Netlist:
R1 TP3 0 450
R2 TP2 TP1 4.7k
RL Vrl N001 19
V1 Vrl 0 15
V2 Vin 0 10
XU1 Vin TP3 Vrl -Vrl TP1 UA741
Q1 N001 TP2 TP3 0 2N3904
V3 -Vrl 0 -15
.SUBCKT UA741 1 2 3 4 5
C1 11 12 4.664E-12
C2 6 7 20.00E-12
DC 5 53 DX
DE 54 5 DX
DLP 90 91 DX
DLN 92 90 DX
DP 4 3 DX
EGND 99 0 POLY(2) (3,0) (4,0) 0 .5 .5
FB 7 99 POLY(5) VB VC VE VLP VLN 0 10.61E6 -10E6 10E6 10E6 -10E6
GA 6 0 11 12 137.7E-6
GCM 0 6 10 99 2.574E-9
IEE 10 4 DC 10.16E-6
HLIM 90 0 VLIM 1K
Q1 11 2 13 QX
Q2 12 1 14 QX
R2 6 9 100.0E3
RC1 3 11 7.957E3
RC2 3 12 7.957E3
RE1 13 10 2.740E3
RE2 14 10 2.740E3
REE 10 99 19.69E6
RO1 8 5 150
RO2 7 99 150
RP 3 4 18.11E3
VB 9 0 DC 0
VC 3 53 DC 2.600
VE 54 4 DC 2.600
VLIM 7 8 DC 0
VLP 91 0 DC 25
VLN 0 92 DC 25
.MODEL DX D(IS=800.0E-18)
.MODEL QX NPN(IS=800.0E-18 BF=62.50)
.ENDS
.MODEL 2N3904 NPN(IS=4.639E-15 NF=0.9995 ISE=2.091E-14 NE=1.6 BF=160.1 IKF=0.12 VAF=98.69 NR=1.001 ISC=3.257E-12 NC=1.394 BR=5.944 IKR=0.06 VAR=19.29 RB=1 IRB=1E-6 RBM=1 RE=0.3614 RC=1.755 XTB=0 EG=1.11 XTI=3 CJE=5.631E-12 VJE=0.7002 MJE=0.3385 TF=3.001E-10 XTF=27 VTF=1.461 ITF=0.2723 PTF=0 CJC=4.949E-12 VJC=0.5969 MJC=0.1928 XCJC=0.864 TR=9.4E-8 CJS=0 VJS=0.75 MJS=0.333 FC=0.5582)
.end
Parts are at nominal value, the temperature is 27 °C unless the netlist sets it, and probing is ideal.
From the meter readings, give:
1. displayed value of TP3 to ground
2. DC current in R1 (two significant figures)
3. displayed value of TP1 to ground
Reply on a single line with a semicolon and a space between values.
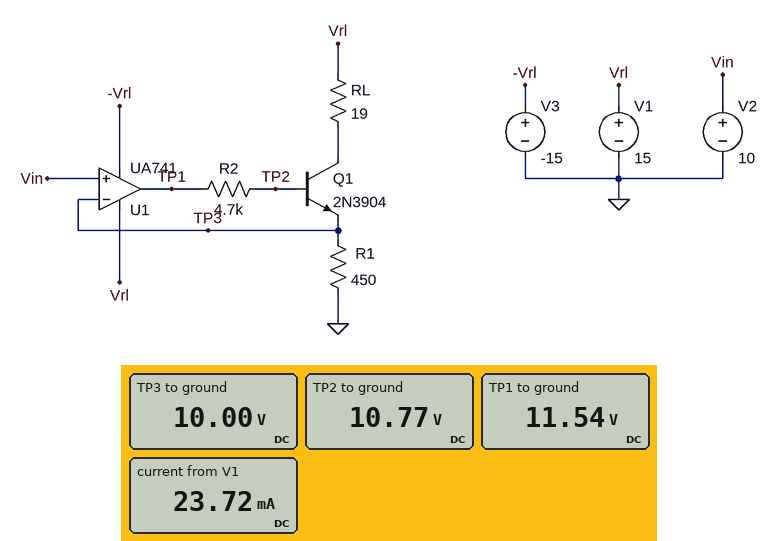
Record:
10.00 V; 22 mA; 11.54 V
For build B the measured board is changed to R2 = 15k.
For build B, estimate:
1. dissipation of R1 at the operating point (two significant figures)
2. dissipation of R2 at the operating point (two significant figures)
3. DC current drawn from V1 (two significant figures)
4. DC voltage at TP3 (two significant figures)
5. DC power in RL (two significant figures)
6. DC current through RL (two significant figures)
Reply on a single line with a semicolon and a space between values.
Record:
210 mW; 390 µW; 23 mA; 9.8 V; 8.9 mW; 22 mA
